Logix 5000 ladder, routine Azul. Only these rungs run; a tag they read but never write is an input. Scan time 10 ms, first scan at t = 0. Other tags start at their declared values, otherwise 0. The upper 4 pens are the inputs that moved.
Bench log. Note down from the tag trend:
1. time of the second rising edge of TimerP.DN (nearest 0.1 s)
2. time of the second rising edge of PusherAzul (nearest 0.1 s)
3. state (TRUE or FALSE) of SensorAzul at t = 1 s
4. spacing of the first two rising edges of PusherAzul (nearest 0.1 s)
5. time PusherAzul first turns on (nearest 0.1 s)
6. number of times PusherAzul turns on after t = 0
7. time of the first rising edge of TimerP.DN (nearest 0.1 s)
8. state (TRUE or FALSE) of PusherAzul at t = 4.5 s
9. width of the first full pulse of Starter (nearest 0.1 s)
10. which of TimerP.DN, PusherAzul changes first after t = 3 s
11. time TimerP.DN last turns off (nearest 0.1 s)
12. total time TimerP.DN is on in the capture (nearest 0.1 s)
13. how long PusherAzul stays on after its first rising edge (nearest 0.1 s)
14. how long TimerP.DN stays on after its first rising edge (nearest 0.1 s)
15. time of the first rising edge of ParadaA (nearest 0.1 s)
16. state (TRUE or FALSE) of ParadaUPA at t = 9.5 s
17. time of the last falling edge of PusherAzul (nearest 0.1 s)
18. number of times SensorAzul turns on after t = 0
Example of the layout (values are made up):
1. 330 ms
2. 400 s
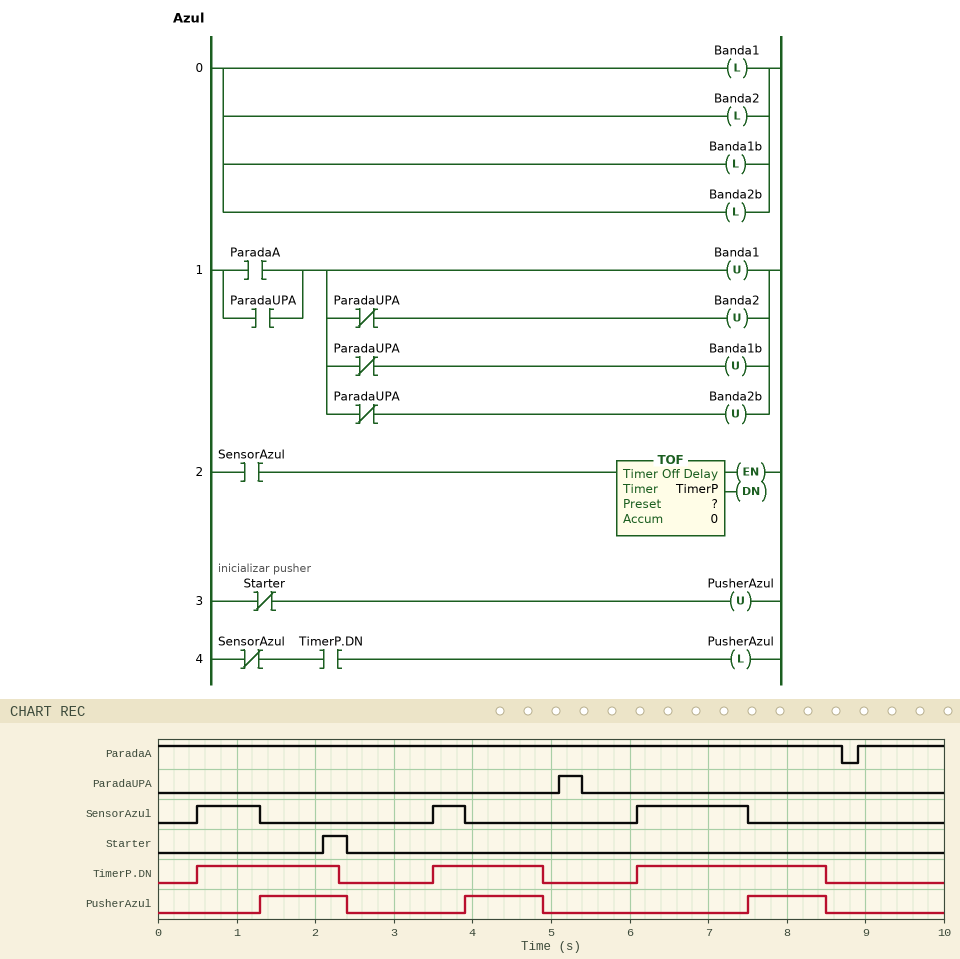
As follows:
1. 3.5 s
2. 3.9 s
3. TRUE
4. 2.6 s
5. 1.3 s
6. 3
7. 0.5 s
8. TRUE
9. 0.3 s
10. TimerP.DN
11. 8.5 s
12. 5.6 s
13. 1.1 s
14. 1.8 s
15. 8.9 s
16. FALSE
17. 8.5 s
18. 3
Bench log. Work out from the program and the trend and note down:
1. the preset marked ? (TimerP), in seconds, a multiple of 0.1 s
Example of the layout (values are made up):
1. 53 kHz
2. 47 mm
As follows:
1. 1.0 s
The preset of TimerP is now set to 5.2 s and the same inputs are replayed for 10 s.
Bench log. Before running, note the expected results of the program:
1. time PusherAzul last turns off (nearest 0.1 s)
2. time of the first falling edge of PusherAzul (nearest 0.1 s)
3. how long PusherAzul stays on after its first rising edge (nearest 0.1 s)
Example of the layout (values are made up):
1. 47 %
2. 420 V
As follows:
1. 6.1 s
2. 3.5 s
3. 2.2 s
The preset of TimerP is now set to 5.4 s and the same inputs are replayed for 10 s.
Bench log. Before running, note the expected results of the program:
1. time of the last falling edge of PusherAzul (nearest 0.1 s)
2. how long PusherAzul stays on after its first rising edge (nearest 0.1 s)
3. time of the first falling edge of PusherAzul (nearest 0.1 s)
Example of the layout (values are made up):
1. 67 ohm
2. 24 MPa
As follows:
1. 6.1 s
2. 2.2 s
3. 3.5 s
